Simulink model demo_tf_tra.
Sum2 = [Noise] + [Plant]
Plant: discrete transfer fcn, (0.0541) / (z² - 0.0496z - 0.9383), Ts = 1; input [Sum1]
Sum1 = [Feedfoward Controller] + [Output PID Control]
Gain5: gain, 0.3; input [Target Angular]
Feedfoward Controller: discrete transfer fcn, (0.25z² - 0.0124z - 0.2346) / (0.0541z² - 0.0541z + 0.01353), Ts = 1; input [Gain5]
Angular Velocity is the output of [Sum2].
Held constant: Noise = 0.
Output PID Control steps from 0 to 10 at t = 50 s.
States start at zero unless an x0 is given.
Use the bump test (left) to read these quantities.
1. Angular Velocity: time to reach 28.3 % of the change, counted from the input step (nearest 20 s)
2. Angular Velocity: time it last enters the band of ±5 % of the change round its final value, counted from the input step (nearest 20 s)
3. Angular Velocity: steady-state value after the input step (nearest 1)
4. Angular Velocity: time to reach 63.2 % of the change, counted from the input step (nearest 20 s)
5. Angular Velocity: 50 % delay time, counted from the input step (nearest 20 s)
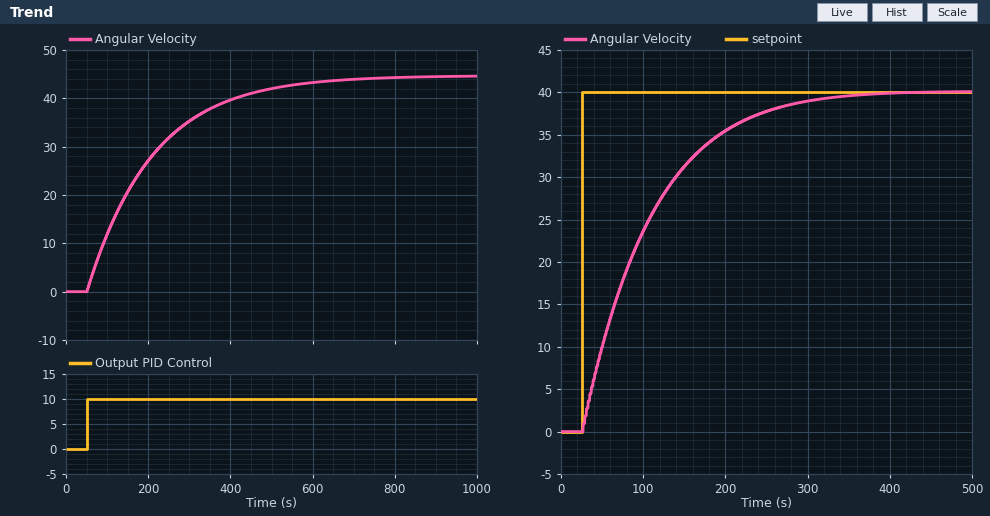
60 s
480 s
45
160 s
120 s
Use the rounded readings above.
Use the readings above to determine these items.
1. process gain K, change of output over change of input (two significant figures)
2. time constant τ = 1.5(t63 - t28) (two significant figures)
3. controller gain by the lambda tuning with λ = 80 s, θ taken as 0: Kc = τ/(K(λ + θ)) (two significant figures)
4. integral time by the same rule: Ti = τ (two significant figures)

4.5
150 s
0.42
150 s
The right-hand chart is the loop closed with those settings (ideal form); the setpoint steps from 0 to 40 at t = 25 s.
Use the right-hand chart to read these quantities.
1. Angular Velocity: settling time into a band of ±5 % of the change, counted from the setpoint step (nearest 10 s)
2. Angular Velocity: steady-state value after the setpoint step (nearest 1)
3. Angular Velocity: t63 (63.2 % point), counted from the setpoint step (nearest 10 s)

230 s
40
80 s
